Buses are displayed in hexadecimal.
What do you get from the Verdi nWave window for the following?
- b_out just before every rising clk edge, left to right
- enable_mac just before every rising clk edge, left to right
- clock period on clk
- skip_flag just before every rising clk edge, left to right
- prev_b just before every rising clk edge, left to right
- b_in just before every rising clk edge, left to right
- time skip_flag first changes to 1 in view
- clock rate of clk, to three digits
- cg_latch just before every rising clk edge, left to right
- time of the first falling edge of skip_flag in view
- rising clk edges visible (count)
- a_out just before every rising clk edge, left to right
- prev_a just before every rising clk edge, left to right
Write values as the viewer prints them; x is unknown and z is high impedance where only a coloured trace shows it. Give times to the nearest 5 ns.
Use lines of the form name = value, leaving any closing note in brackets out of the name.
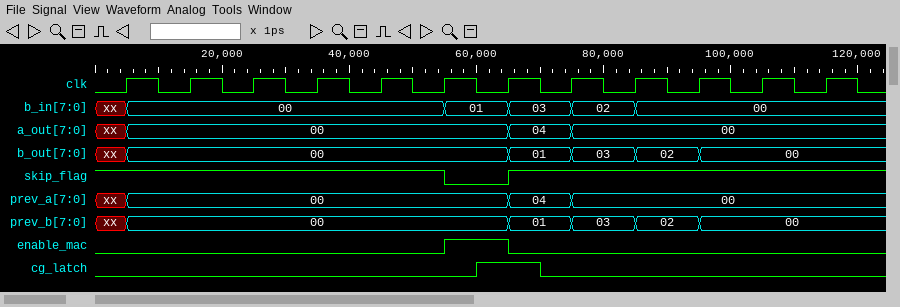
b_out just before every rising clk edge, left to right = xx, 00, 00, 00, 00, 00, 00, 01, 03, 02, 00, 00
enable_mac just before every rising clk edge, left to right = 0 0 0 0 0 0 1 0 0 0 0 0
clock period on clk = 10 ns
skip_flag just before every rising clk edge, left to right = 1 1 1 1 1 1 0 1 1 1 1 1
prev_b just before every rising clk edge, left to right = xx, 00, 00, 00, 00, 00, 00, 01, 03, 02, 00, 00
b_in just before every rising clk edge, left to right = xx, 00, 00, 00, 00, 00, 01, 03, 02, 00, 00, 00
time skip_flag first changes to 1 in view = 65 ns
clock rate of clk, to three digits = 100 MHz
cg_latch just before every rising clk edge, left to right = 0 0 0 0 0 0 1 0 0 0 0 0
time of the first falling edge of skip_flag in view = 55 ns
rising clk edges visible = 12
a_out just before every rising clk edge, left to right = xx, 00, 00, 00, 00, 00, 00, 04, 00, 00, 00, 00
prev_a just before every rising clk edge, left to right = xx, 00, 00, 00, 00, 00, 00, 04, 00, 00, 00, 00
